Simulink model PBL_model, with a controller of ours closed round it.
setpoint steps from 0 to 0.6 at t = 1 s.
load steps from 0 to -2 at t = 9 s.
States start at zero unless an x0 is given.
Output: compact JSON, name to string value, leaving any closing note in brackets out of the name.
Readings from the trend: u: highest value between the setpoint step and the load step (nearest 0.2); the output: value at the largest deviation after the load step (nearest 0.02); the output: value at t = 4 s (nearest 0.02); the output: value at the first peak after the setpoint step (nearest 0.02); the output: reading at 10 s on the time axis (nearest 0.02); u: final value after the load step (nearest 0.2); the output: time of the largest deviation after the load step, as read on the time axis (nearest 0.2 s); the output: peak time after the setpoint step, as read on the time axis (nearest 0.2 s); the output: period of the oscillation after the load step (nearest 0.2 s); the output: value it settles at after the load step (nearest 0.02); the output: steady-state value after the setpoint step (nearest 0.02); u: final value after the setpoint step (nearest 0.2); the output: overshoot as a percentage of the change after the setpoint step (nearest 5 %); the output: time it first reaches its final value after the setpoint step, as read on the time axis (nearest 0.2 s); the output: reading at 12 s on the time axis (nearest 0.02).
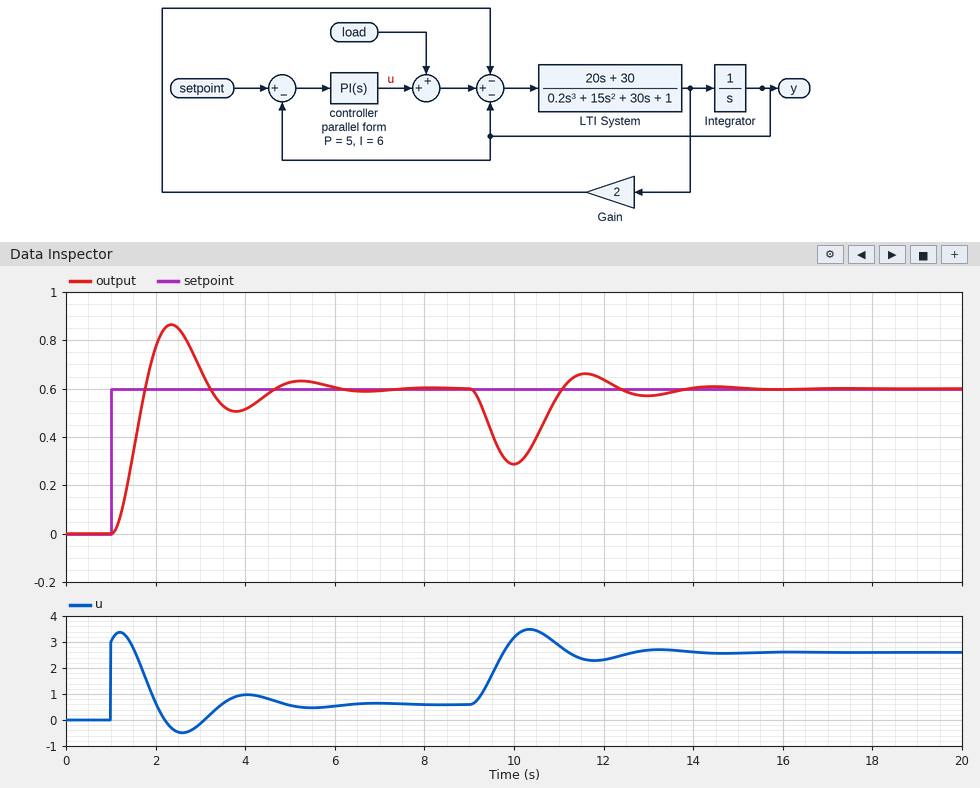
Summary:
{"u: highest value between the setpoint step and the load step": "3.4", "the output: value at the largest deviation after the load step": "0.28", "the output: value at t = 4 s": "0.52", "the output: value at the first peak after the setpoint step": "0.86", "the output: reading at 10 s on the time axis": "0.28", "u: final value after the load step": "2.6", "the output: time of the largest deviation after the load step, as read on the time axis": "10.0 s", "the output: peak time after the setpoint step, as read on the time axis": "2.4 s", "the output: period of the oscillation after the load step": "3.0 s", "the output: value it settles at after the load step": "0.60", "the output: steady-state value after the setpoint step": "0.60", "u: final value after the setpoint step": "0.6", "the output: overshoot as a percentage of the change after the setpoint step": "45 %", "the output: time it first reaches its final value after the setpoint step, as read on the time axis": "1.8 s", "the output: reading at 12 s on the time axis": "0.64"}
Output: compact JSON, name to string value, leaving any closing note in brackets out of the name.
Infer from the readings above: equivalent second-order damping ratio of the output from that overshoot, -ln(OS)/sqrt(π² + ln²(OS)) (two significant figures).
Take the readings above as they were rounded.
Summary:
{"equivalent second-order damping ratio of the output from that overshoot, -ln(OS)/sqrt(π² + ln²(OS))": "0.25"}
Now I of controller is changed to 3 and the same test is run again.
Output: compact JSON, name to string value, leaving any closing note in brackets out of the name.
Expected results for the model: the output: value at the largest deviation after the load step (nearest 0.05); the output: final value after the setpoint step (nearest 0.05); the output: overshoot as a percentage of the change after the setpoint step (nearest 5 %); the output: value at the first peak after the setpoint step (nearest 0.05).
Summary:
{"the output: value at the largest deviation after the load step": "0.25", "the output: final value after the setpoint step": "0.60", "the output: overshoot as a percentage of the change after the setpoint step": "25 %", "the output: value at the first peak after the setpoint step": "0.75"}
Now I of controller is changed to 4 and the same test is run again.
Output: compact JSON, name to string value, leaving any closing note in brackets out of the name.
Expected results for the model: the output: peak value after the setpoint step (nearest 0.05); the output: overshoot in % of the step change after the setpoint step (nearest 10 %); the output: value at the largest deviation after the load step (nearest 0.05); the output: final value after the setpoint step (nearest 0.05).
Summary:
{"the output: peak value after the setpoint step": "0.80", "the output: overshoot in % of the step change after the setpoint step": "30 %", "the output: value at the largest deviation after the load step": "0.25", "the output: final value after the setpoint step": "0.60"}
